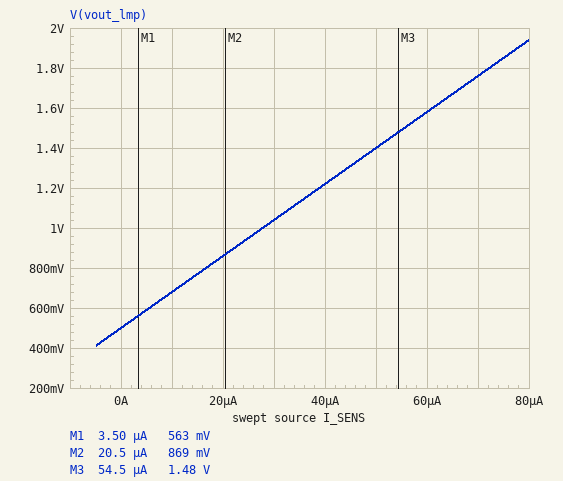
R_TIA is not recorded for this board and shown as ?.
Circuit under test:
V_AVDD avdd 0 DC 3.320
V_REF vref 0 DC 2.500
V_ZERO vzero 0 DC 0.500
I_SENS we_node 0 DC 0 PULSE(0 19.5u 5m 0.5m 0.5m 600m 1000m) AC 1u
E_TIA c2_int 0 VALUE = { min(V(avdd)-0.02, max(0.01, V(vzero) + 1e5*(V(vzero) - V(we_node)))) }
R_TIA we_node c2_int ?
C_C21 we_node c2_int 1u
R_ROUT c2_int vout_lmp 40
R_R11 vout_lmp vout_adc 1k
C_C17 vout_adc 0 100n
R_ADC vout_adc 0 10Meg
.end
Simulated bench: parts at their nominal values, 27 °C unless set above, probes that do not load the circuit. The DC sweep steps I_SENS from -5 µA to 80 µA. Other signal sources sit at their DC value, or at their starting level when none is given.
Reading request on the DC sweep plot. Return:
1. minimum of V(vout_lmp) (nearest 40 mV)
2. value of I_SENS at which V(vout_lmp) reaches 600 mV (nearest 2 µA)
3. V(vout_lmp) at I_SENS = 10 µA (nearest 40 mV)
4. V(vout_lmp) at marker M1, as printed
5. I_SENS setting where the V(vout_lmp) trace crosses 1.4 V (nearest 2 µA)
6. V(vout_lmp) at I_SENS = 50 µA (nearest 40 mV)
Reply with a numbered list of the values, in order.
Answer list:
1. 400 mV
2. 6 µA
3. 680 mV
4. 563 mV
5. 50 µA
6. 1.40 V
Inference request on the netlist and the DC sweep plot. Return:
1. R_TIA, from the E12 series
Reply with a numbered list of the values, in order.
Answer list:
1. 18 kΩ
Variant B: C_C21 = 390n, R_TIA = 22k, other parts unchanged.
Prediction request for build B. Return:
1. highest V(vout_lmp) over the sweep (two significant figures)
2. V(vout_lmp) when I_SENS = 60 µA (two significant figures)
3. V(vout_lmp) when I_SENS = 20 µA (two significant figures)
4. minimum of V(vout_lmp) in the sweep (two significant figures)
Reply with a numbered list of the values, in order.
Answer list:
1. 2.3 V
2. 1.8 V
3. 940 mV
4. 390 mV
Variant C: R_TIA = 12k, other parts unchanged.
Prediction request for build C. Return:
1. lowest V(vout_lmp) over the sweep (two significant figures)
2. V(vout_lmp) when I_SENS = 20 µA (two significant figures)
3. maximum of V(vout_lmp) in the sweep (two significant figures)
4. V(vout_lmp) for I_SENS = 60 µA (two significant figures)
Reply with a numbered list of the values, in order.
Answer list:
1. 440 mV
2. 740 mV
3. 1.5 V
4. 1.2 V
